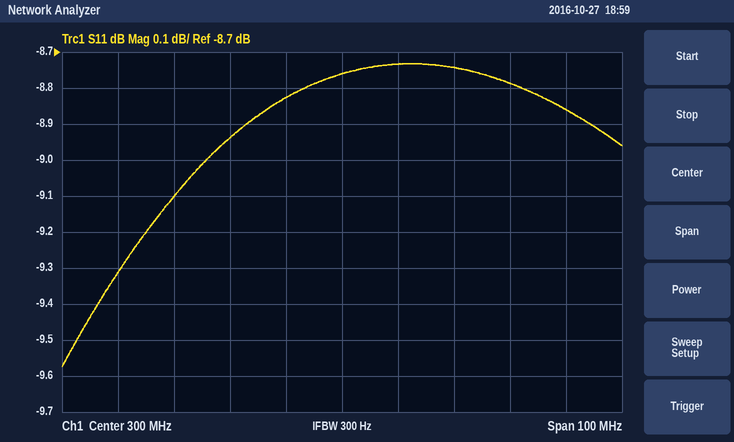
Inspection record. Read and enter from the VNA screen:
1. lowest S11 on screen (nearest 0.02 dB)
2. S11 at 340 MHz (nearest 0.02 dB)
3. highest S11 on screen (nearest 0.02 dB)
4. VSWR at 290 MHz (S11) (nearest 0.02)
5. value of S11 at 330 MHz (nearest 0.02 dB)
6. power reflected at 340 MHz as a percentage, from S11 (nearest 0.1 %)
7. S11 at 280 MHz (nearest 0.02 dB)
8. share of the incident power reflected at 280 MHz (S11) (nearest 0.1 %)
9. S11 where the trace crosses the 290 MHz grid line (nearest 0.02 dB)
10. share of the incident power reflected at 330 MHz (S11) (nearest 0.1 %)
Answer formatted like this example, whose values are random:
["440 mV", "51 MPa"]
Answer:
["-9.58 dB", "-8.86 dB", "-8.74 dB", "2.14", "-8.78 dB", "13.0 %", "-8.94 dB", "12.8 %", "-8.82 dB", "13.2 %"]
